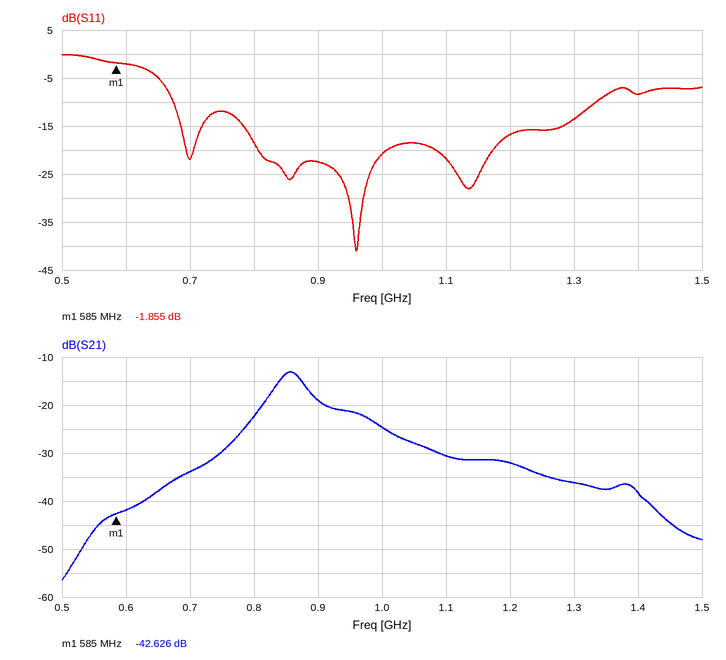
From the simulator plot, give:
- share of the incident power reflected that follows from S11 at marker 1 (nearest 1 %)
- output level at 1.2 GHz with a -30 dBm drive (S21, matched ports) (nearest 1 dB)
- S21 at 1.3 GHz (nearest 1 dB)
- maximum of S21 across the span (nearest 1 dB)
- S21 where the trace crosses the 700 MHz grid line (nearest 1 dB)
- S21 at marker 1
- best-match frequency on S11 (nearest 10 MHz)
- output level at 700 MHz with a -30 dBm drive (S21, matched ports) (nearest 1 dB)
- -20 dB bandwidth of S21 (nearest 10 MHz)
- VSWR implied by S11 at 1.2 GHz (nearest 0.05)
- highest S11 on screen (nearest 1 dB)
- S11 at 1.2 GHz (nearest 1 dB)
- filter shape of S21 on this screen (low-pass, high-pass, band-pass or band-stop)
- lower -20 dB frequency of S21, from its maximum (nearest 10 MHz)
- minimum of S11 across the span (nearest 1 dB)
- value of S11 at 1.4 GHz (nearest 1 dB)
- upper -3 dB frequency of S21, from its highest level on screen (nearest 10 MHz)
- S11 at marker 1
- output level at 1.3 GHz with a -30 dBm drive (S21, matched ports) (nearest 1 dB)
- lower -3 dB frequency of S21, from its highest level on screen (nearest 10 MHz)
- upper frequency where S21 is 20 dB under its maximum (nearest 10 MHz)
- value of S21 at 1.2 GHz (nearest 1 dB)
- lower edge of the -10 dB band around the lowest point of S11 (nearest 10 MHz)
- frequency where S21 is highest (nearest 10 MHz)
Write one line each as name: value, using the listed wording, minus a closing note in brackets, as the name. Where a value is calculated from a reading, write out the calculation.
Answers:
share of the incident power reflected that follows from S11 at marker 1: 10^(-1.855/10) ≈ 65 %
output level at 1.2 GHz with a -30 dBm drive (S21, matched ports): -30 dBm + (-32 dB) = -62 dBm
S21 at 1.3 GHz: -36 dB
maximum of S21 across the span: -13 dB
S21 where the trace crosses the 700 MHz grid line: -34 dB
S21 at marker 1: -42.626 dB
best-match frequency on S11: 960 MHz
output level at 700 MHz with a -30 dBm drive (S21, matched ports): -30 dBm + (-34 dB) = -64 dBm
-20 dB bandwidth of S21: 1.22 GHz − 710 MHz = 510 MHz
VSWR implied by S11 at 1.2 GHz: |Γ| = 10^(-17/20) = 0.1413; VSWR = (1 + 0.1413)/(1 − 0.1413) ≈ 1.33, so 1.35 to the nearest 0.05
highest S11 on screen: 0 dB
S11 at 1.2 GHz: -17 dB
filter shape of S21 on this screen: band-pass
lower -20 dB frequency of S21, from its maximum: 710 MHz
minimum of S11 across the span: -41 dB
value of S11 at 1.4 GHz: -8 dB
upper -3 dB frequency of S21, from its highest level on screen: 880 MHz
S11 at marker 1: -1.855 dB
output level at 1.3 GHz with a -30 dBm drive (S21, matched ports): -30 dBm + (-36 dB) = -66 dBm
lower -3 dB frequency of S21, from its highest level on screen: 830 MHz
upper frequency where S21 is 20 dB under its maximum: 1.22 GHz
value of S21 at 1.2 GHz: -32 dB
lower edge of the -10 dB band around the lowest point of S11: 670 MHz
frequency where S21 is highest: 860 MHz
